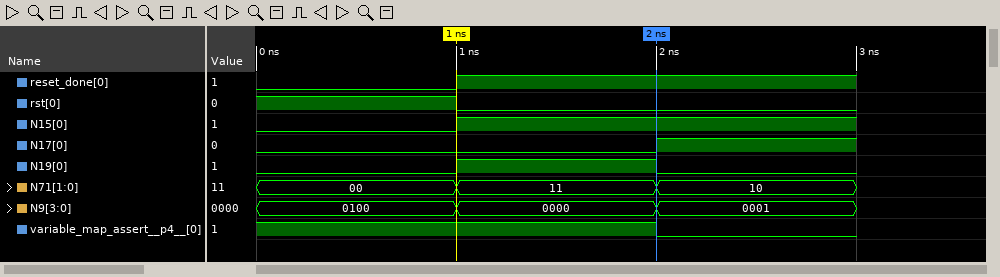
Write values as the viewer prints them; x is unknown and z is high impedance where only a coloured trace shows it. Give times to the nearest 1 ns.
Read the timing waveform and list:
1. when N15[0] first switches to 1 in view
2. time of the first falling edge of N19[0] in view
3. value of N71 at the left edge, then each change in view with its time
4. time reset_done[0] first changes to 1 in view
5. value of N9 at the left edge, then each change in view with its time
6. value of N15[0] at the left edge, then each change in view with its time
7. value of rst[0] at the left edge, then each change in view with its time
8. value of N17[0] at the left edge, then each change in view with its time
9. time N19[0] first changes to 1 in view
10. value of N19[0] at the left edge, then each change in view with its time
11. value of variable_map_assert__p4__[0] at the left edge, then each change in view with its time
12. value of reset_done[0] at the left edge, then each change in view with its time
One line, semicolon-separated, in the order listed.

1 ns; 2 ns; 00, 11 at 1 ns, 10 at 2 ns; 1 ns; 0100, 0000 at 1 ns, 0001 at 2 ns; 0, 1 at 1 ns; 1, 0 at 1 ns; 0, 1 at 2 ns; 1 ns; 0, 1 at 1 ns, 0 at 2 ns; 1, 0 at 2 ns; 0, 1 at 1 ns
